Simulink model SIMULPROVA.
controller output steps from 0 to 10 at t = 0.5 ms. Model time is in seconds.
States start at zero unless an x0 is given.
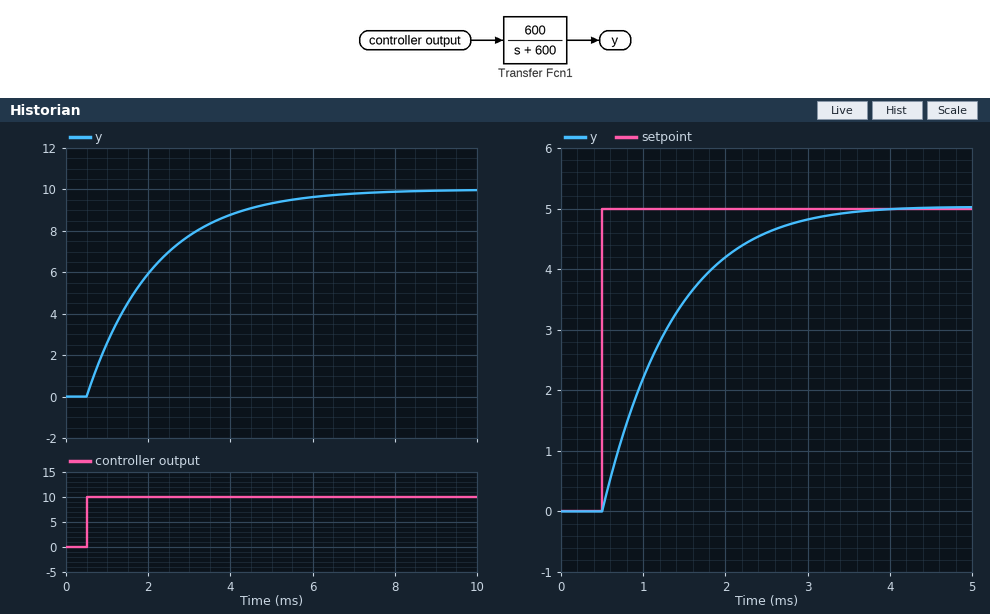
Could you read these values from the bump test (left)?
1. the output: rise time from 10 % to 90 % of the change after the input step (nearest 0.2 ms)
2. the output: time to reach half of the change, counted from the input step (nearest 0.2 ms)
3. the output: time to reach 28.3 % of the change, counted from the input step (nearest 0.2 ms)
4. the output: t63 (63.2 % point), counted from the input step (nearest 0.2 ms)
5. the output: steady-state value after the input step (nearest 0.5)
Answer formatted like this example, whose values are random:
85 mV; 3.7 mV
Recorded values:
3.6 ms; 1.2 ms; 0.6 ms; 1.6 ms; 10.0
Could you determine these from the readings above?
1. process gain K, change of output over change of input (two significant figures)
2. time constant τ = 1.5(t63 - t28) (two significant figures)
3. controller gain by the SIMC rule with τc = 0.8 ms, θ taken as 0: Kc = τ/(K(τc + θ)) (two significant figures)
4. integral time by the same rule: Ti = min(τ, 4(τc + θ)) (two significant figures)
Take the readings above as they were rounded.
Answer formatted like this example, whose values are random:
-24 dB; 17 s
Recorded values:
1.0; 1.5 ms; 1.9; 1.5 ms
